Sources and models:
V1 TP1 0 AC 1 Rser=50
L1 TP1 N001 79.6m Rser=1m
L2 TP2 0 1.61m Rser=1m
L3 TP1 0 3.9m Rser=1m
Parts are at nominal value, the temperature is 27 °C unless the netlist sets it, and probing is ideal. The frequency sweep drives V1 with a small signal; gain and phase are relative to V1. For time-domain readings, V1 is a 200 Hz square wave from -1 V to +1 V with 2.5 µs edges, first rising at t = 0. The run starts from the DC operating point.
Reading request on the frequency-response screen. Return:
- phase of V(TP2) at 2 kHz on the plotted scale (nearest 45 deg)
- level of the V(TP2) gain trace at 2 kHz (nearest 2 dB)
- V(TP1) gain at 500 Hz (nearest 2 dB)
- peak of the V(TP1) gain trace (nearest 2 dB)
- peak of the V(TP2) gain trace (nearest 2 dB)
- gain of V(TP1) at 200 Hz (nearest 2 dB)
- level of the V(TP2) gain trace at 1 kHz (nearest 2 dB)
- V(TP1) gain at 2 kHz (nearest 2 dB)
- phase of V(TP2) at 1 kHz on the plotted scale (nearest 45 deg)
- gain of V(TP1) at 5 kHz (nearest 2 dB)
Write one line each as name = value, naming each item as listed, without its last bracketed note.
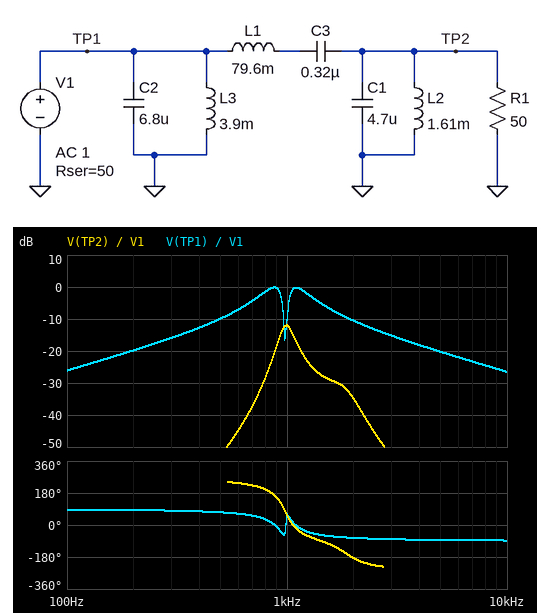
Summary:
phase of V(TP2) at 2 kHz on the plotted scale = -180 deg
level of the V(TP2) gain trace at 2 kHz = -34 dB
V(TP1) gain at 500 Hz = -10 dB
peak of the V(TP1) gain trace = 0 dB
peak of the V(TP2) gain trace = -12 dB
gain of V(TP1) at 200 Hz = -20 dB
level of the V(TP2) gain trace at 1 kHz = -12 dB
V(TP1) gain at 2 kHz = -10 dB
phase of V(TP2) at 1 kHz on the plotted scale = 45 deg
gain of V(TP1) at 5 kHz = -20 dB
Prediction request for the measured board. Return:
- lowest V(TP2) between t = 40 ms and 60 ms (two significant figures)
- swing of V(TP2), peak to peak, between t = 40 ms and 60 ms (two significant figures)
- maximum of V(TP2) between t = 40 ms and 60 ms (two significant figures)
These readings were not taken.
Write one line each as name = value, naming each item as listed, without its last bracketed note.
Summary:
lowest V(TP2) between t = 40 ms and 60 ms = -74 mV
swing of V(TP2), peak to peak, between t = 40 ms and 60 ms = 150 mV
maximum of V(TP2) between t = 40 ms and 60 ms = 74 mV
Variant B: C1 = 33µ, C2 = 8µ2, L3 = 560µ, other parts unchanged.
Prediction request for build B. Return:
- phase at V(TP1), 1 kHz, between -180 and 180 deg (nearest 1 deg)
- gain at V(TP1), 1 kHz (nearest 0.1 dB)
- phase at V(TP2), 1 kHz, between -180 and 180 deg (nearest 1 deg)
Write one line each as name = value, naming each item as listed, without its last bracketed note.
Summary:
phase at V(TP1), 1 kHz, between -180 and 180 deg = 53 deg
gain at V(TP1), 1 kHz = -14.1 dB
phase at V(TP2), 1 kHz, between -180 and 180 deg = 48 deg
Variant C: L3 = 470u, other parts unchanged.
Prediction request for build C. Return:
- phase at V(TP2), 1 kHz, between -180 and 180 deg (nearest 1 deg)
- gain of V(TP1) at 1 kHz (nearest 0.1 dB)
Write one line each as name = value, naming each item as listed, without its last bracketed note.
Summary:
phase at V(TP2), 1 kHz, between -180 and 180 deg = 82 deg
gain of V(TP1) at 1 kHz = -25.0 dB
